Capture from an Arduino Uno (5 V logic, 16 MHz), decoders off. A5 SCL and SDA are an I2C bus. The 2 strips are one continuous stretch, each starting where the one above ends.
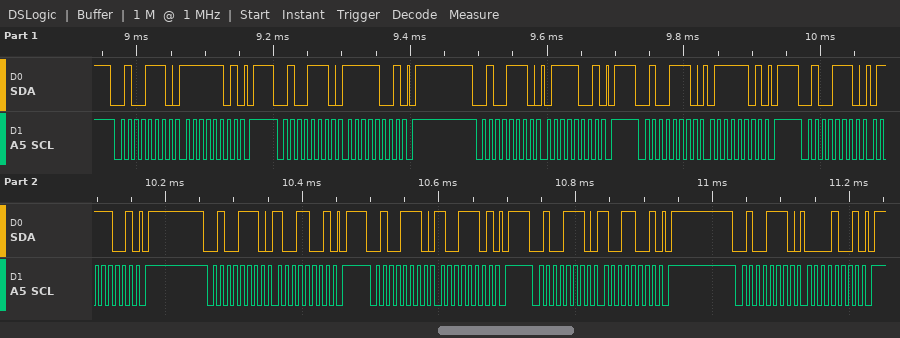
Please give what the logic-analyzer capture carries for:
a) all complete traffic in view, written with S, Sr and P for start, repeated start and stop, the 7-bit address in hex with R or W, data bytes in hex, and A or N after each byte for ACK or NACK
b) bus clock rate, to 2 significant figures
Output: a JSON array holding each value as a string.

["S 27W A FD A P S 27W A F9 A P S 27W A 79 A P S 27W A 7D A P S 27W A 79 A P S 27W A 99 A P S 27W A 9D A P S 27W A 99 A P S 27W A 09 A P", "100 kHz"]
